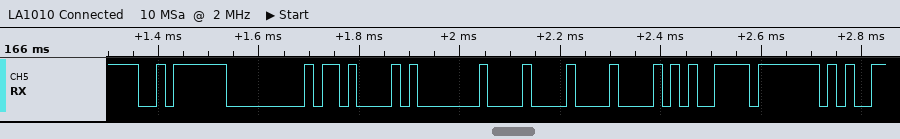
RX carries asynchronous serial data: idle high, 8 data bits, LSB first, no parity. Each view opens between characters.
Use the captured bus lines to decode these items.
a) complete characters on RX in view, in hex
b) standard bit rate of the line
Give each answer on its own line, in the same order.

FA, 00, 0B, 01, 08, 08, E5, 7F
57600 baud
